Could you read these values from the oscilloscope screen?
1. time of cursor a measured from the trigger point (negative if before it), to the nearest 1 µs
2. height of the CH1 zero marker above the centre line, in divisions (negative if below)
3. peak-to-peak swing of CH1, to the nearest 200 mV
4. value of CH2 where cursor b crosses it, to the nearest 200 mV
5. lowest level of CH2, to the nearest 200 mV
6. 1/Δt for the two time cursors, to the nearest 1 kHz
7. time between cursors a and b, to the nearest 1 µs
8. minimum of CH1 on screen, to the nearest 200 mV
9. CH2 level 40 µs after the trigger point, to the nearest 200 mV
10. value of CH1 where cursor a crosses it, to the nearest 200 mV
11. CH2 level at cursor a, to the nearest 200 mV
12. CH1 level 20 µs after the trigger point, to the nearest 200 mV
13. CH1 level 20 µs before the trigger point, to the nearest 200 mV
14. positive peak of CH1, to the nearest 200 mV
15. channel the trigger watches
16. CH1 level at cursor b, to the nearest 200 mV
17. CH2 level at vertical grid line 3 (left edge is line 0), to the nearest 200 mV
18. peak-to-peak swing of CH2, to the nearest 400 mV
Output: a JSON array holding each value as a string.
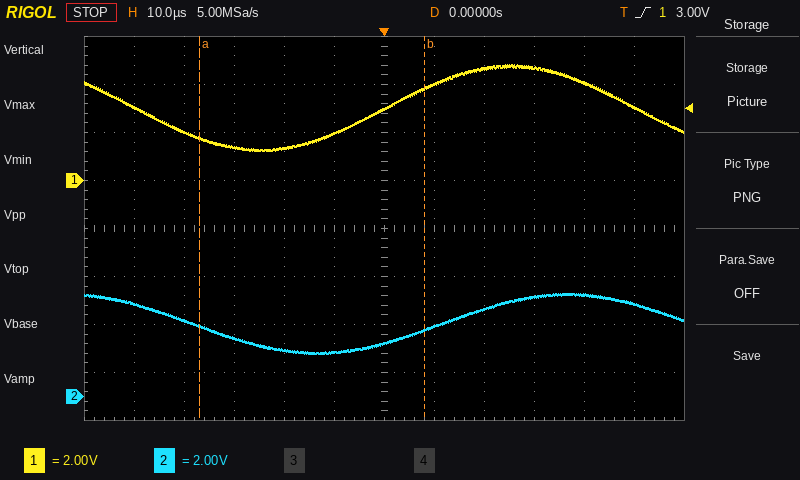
["-37 µs", "+1.0 div", "3.6 V", "2.8 V", "1.8 V", "22 kHz", "45 µs", "1.2 V", "4.2 V", "1.8 V", "3.0 V", "4.6 V", "1.4 V", "4.8 V", "CH1", "3.8 V", "2.4 V", "2.4 V"]
